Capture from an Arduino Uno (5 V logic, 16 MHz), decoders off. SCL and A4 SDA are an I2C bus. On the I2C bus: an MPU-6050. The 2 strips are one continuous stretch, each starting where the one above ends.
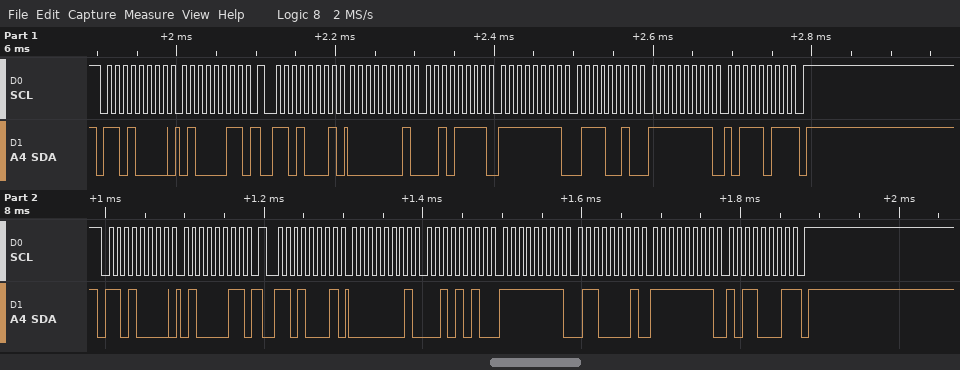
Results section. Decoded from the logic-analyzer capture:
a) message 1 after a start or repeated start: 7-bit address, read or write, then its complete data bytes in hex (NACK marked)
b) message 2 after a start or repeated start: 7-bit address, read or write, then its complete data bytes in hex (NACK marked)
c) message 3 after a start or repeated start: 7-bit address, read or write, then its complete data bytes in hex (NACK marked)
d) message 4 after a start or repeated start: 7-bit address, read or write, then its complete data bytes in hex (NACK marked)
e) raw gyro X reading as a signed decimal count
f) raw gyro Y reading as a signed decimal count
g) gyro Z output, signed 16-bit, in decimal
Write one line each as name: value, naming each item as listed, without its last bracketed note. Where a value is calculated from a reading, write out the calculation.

message 1 after a start or repeated start: 7-bit address, read or write, then its complete data bytes in hex: 0x68 write: 43
message 2 after a start or repeated start: 7-bit address, read or write, then its complete data bytes in hex: 0x68 read: 01 2F FF 72 FF BB NACK
message 3 after a start or repeated start: 7-bit address, read or write, then its complete data bytes in hex: 0x68 write: 43
message 4 after a start or repeated start: 7-bit address, read or write, then its complete data bytes in hex: 0x68 read: 01 2A FF 61 FF B1 NACK
raw gyro X reading as a signed decimal count: 0x012F = 303
raw gyro Y reading as a signed decimal count: 0xFF72 = -142
gyro Z output, signed 16-bit, in decimal: 0xFFBB = -69
